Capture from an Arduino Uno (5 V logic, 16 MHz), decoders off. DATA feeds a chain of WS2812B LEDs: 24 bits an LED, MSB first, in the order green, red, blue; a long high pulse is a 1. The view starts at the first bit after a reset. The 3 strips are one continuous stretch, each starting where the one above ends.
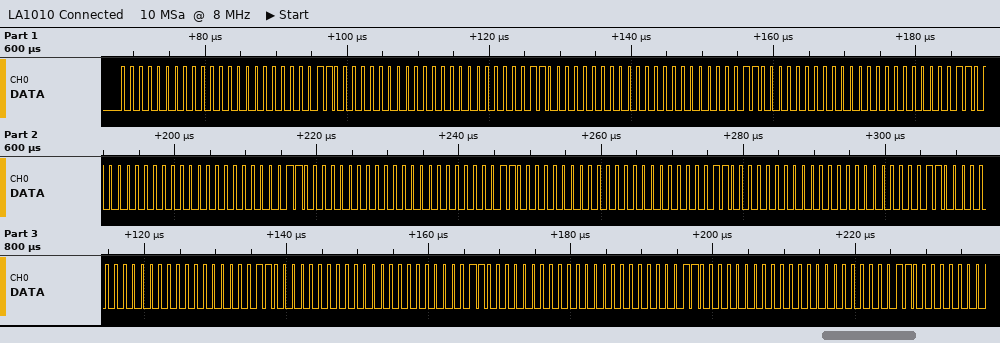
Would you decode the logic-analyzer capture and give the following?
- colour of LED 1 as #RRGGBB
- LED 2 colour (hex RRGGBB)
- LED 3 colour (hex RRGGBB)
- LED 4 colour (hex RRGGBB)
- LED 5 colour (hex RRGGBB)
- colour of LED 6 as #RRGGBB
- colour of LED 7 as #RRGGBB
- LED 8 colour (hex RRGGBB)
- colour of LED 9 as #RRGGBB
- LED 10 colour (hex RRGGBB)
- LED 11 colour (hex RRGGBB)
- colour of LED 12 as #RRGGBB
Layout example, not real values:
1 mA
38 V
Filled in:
#000003
#000003
#000003
#000003
#000003
#000003
#000003
#000003
#000003
#000003
#000003
#000003
